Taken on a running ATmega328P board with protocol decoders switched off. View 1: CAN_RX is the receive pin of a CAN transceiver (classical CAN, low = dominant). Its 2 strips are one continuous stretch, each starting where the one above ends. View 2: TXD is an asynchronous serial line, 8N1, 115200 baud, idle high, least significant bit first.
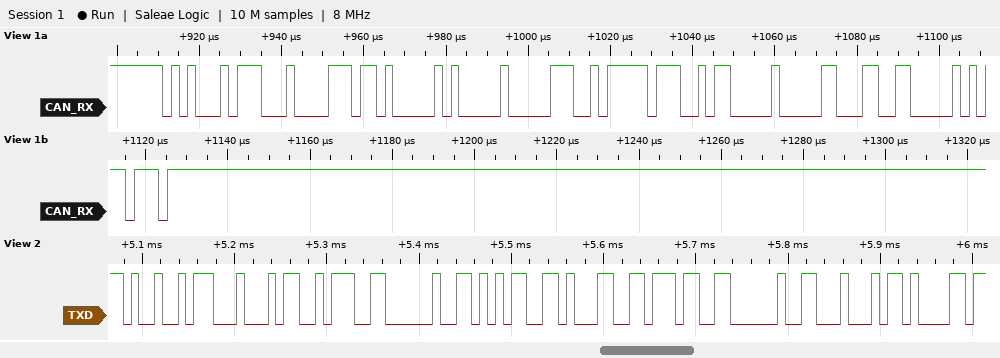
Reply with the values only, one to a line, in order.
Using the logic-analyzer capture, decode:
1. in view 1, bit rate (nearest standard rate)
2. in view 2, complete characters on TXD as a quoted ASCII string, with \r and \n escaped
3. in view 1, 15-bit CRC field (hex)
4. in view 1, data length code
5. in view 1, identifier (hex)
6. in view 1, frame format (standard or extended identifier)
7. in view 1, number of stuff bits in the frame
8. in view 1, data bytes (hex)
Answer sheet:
500 kbit/s
"ID: 517 Da"
0x605B
8
0x517
standard
7
76 81 00 32 FF 2C 00 8C
